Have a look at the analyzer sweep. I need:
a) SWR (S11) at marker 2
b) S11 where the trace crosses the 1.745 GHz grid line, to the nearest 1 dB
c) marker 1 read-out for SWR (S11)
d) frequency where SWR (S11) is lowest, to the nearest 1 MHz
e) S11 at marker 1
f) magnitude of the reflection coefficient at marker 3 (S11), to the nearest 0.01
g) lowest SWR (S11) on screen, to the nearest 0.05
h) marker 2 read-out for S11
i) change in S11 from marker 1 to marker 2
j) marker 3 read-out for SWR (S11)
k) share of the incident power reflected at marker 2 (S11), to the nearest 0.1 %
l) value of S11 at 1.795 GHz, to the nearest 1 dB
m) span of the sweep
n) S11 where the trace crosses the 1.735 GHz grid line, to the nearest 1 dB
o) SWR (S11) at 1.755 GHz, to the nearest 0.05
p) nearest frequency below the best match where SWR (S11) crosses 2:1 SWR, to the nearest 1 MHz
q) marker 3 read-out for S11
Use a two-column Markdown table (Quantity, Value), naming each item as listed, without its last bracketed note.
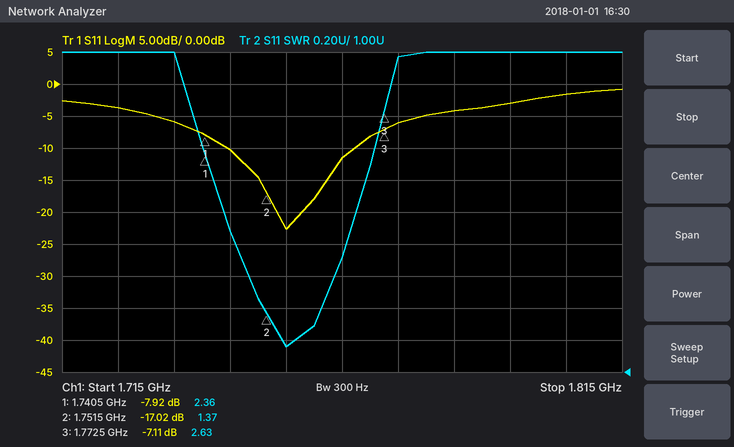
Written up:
| Quantity | Value |
|---|---|
| SWR (S11) at marker 2 | 1.37 |
| S11 where the trace crosses the 1.745 GHz grid line, to the nearest 1 dB | -10 dB |
| marker 1 read-out for SWR | 2.36 |
| frequency where SWR (S11) is lowest, to the nearest 1 MHz | 1.755 GHz |
| S11 at marker 1 | -7.92 dB |
| magnitude of the reflection coefficient at marker 3 (S11), to the nearest 0.01 | 0.44 |
| lowest SWR (S11) on screen, to the nearest 0.05 | 1.15 |
| marker 2 read-out for S11 | -17.02 dB |
| change in S11 from marker 1 to marker 2 | -9.10 dB |
| marker 3 read-out for SWR | 2.63 |
| share of the incident power reflected at marker 2 (S11), to the nearest 0.1 % | 2.0 % |
| value of S11 at 1.795 GHz, to the nearest 1 dB | -3 dB |
| span of the sweep | 100 MHz |
| S11 where the trace crosses the 1.735 GHz grid line, to the nearest 1 dB | -6 dB |
| SWR (S11) at 1.755 GHz, to the nearest 0.05 | 1.15 |
| nearest frequency below the best match where SWR (S11) crosses 2:1 SWR, to the nearest 1 MHz | 1.744 GHz |
| marker 3 read-out for S11 | -7.11 dB |
